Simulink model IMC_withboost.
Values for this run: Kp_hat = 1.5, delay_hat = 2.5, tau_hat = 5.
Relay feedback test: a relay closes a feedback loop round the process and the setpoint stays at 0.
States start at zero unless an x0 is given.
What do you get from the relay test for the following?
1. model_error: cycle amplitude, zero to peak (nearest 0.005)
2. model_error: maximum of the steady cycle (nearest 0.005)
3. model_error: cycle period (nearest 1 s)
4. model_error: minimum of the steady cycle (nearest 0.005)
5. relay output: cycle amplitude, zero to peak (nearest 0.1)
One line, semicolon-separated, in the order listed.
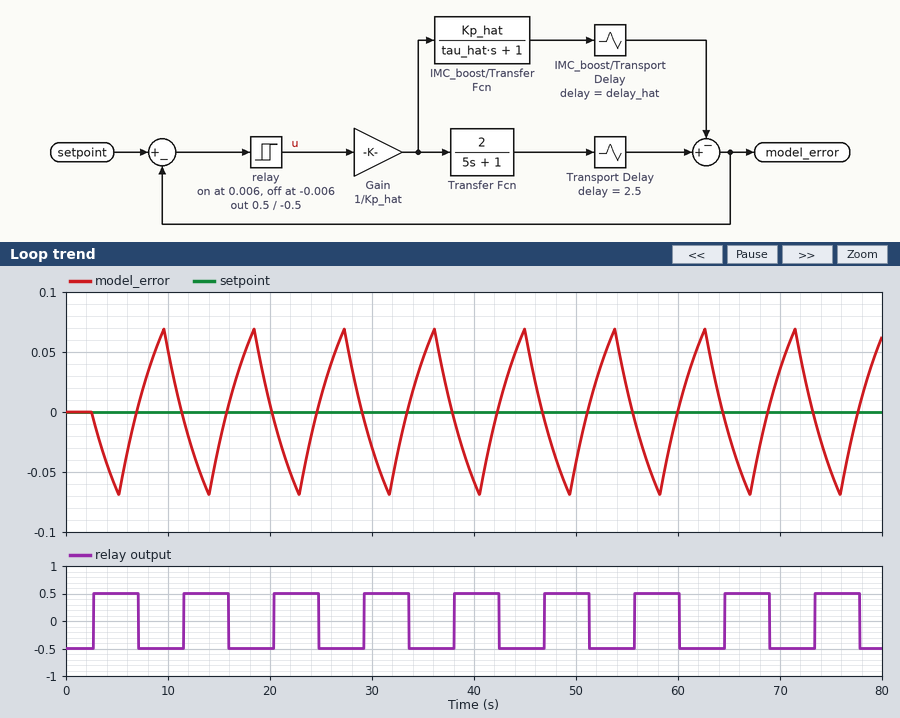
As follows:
0.070; 0.070; 9 s; -0.070; 0.5
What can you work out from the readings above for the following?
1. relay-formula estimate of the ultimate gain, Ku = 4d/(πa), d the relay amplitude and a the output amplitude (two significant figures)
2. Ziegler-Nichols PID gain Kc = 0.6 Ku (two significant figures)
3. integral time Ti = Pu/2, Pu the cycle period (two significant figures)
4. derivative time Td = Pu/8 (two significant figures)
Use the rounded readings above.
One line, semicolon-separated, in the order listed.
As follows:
9.1; 5.5; 4.5 s; 1.1 s
